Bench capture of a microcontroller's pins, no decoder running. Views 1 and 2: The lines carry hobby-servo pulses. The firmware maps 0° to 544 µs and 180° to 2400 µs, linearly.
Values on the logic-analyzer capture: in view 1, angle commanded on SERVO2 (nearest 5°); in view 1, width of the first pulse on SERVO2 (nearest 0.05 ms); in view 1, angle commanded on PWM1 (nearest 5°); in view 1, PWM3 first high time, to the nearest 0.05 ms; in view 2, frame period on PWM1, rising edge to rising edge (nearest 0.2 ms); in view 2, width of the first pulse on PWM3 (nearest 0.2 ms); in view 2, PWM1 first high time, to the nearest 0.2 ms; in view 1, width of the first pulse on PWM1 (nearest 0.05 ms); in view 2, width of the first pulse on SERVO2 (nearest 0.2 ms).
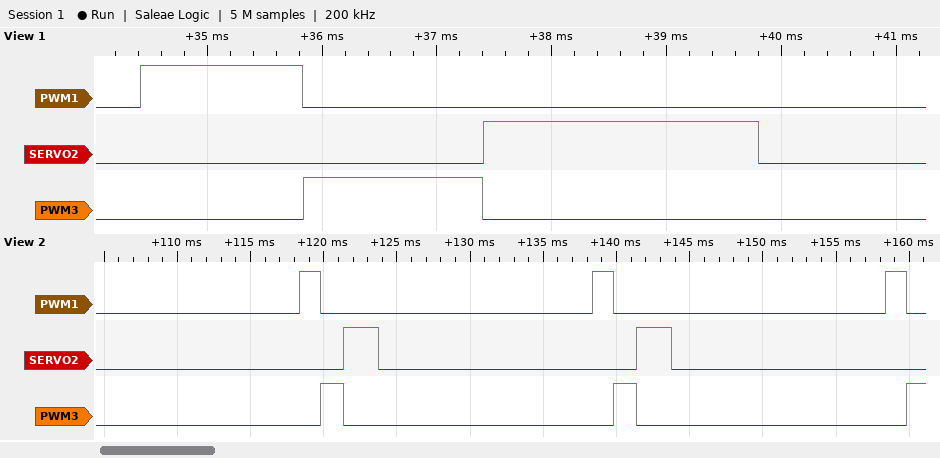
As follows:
180°
2.40 ms
85°
1.55 ms
20.0 ms
1.6 ms
1.4 ms
1.40 ms
2.4 ms
